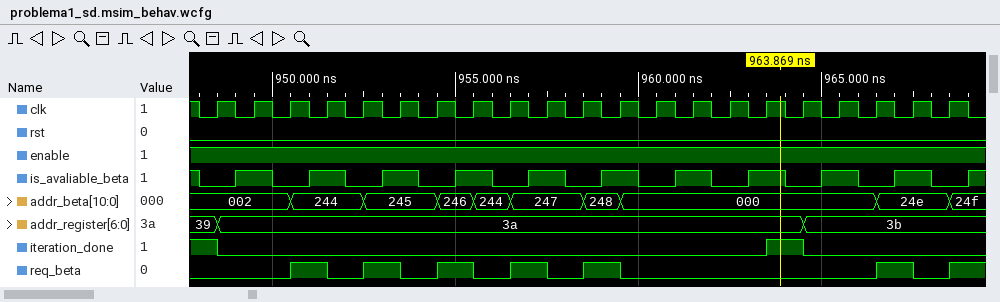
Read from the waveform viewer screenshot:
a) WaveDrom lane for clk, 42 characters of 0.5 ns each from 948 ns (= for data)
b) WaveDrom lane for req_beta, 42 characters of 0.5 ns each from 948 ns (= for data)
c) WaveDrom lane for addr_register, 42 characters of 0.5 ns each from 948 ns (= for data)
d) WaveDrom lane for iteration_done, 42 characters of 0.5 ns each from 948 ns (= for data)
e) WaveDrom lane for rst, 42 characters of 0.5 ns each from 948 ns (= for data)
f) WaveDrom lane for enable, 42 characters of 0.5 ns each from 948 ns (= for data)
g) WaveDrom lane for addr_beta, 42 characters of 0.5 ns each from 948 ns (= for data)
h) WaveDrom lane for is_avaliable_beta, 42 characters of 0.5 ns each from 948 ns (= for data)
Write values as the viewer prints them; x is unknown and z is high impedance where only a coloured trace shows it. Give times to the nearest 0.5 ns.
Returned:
{name: 'clk', wave: '010101010101010101010101010101010101010101'}
{name: 'req_beta', wave: '0....1.0.1.0.1.0.1.0.1.0.............1.0.1'}
{name: 'addr_register', wave: '==...............................=........', data: '39 3a 3b'}
{name: 'iteration_done', wave: '10.............................1.0........'}
{name: 'rst', wave: '0.........................................'}
{name: 'enable', wave: '1.........................................'}
{name: 'addr_beta', wave: '=....=...=...=.=.=...=.=.............=...=', data: '002 244 245 246 244 247 248 000 24e 24f'}
{name: 'is_avaliable_beta', wave: '0.1.0.1.0.1.0.1.0.1.0.1.0.1.0.1.0.1.0.1.0.'}
